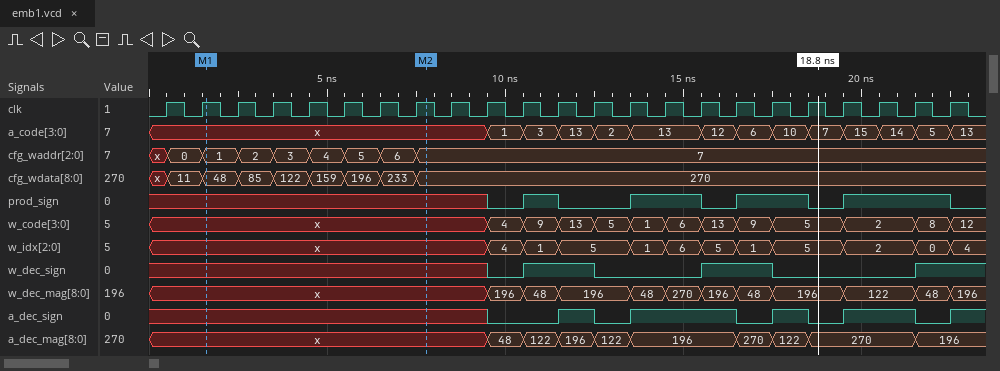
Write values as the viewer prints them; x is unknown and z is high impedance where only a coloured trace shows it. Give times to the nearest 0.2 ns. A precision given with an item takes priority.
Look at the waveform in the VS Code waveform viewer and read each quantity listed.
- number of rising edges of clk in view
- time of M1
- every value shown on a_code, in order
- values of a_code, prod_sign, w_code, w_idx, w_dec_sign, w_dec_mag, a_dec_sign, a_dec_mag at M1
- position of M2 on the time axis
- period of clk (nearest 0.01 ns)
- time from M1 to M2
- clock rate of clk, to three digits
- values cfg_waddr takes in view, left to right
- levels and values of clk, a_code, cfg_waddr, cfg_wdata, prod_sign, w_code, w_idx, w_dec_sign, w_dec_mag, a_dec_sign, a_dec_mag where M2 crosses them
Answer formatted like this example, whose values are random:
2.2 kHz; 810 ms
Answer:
23; 1.6 ns; x, 1, 3, 13, 2, 13, 12, 6, 10, 7, 15, 14, 5, 13; a_code=x, prod_sign=x, w_code=x, w_idx=x, w_dec_sign=x, w_dec_mag=x, a_dec_sign=x, a_dec_mag=x; 7.8 ns; 1 ns; 6.2 ns; 1.00 GHz; x, 0, 1, 2, 3, 4, 5, 6, 7; clk=1, a_code=x, cfg_waddr=7, cfg_wdata=270, prod_sign=x, w_code=x, w_idx=x, w_dec_sign=x, w_dec_mag=x, a_dec_sign=x, a_dec_mag=x
